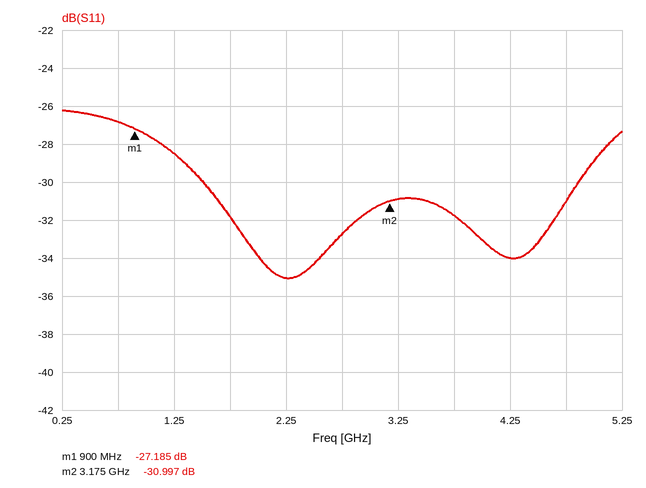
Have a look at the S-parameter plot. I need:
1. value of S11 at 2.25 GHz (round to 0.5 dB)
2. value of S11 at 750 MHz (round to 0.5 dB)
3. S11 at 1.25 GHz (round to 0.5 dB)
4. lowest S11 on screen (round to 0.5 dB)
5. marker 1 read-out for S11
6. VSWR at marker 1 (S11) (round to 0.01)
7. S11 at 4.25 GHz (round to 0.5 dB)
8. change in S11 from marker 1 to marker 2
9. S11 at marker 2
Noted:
-35.0 dB
-27.0 dB
-28.5 dB
-35.0 dB
-27.185 dB
1.09
-34.0 dB
-3.812 dB
-30.997 dB
